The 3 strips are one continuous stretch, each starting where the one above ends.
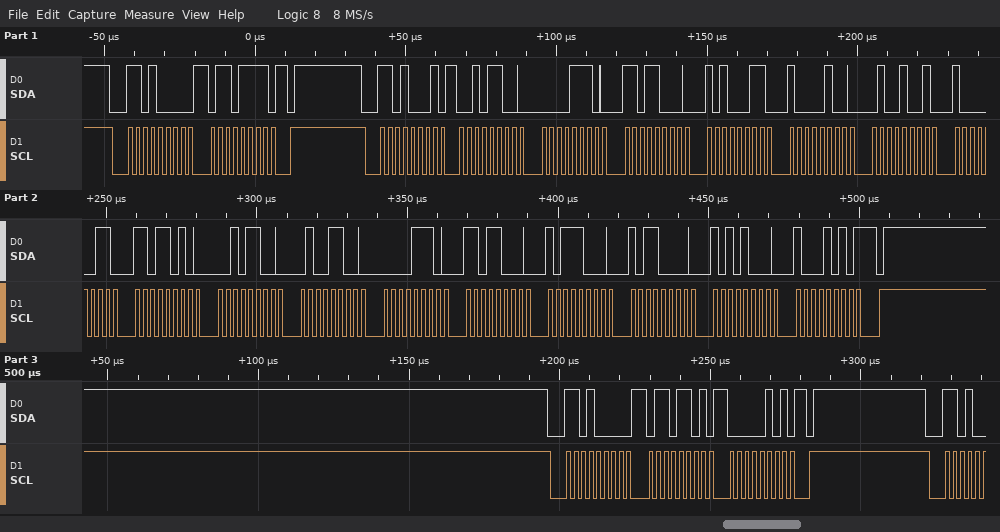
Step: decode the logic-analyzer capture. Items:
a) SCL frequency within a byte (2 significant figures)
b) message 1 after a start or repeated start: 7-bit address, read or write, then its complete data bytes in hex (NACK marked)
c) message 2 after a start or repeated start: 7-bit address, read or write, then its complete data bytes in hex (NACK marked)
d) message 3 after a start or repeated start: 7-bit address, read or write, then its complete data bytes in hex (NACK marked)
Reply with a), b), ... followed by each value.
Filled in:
a) 400 kHz
b) 0x68 write: 6F
c) 0x68 read: 2C 0E D8 A3 84 49 83 DA 2C 4C 0E D8 B8 B0 A8 8A NACK
d) 0x68 write: 6D 05
